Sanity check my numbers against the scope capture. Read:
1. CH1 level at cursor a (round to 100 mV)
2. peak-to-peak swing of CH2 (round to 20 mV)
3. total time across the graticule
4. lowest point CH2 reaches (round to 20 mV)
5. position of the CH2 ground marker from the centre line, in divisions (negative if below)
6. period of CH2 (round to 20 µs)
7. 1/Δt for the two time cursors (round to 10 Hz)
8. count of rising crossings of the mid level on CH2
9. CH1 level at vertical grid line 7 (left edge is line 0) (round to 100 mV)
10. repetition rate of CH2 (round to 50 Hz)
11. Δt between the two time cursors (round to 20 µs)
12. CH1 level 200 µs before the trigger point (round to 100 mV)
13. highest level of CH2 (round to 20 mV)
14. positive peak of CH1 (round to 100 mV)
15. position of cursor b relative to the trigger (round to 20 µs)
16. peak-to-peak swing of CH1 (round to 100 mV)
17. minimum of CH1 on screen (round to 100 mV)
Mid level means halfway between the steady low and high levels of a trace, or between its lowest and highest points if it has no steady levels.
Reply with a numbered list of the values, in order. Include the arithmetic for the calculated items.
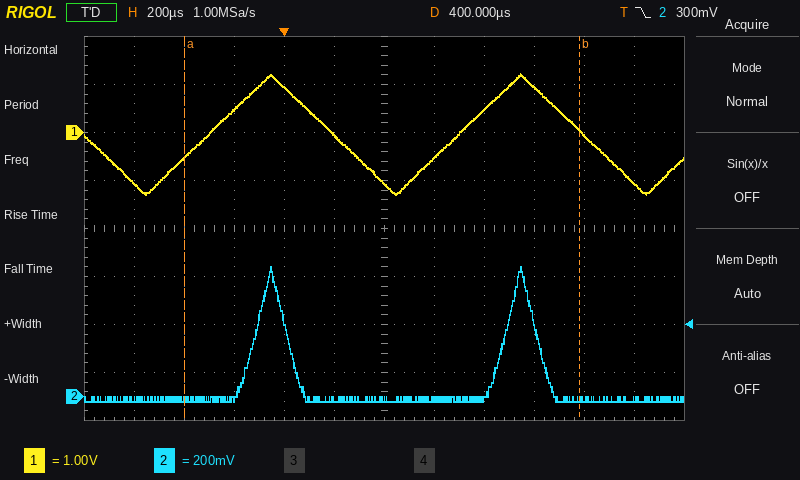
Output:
1. -500 mV
2. 540 mV − (-20 mV) = 560 mV
3. 2.4 ms
4. -20 mV
5. -3.5 div
6. 1.00 ms
7. 1 / 1.58 ms ≈ 630 Hz
8. 2
9. -500 mV
10. 1 / 1.00 ms ≈ 1.00 kHz
11. 1.58 ms
12. 500 mV
13. 540 mV
14. 1.2 V
15. +1.18 ms
16. 1.2 V − (-1.3 V) = 2.5 V
17. -1.3 V
